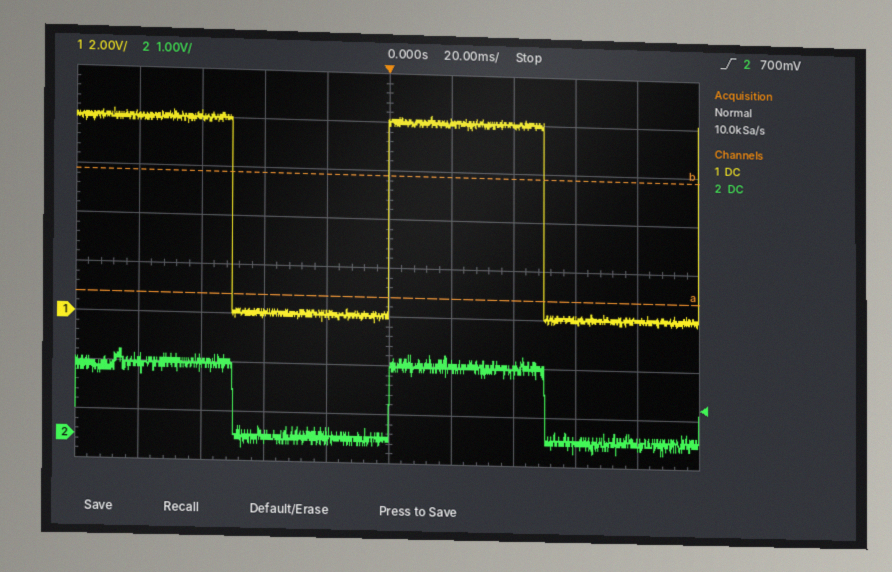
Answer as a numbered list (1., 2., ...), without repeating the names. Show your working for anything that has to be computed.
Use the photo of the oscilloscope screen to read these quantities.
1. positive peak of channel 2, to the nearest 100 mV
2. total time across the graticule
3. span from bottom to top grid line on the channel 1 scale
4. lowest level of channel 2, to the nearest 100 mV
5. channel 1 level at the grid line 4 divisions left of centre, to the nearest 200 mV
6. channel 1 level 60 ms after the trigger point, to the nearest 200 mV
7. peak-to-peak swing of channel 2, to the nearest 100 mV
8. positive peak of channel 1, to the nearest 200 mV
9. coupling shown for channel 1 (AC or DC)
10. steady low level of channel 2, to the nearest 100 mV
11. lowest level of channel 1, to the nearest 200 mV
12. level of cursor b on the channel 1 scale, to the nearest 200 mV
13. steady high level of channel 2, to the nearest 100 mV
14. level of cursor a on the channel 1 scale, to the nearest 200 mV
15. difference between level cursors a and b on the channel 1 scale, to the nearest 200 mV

1. 1.7 V
2. 200 ms
3. 16 V
4. -200 mV
5. 8.0 V
6. 0.0 V
7. 1.7 V − (-200 mV) = 1.9 V
8. 8.2 V
9. DC
10. 0.0 V
11. -200 mV
12. 5.8 V
13. 1.5 V
14. 800 mV
15. 5.0 V
